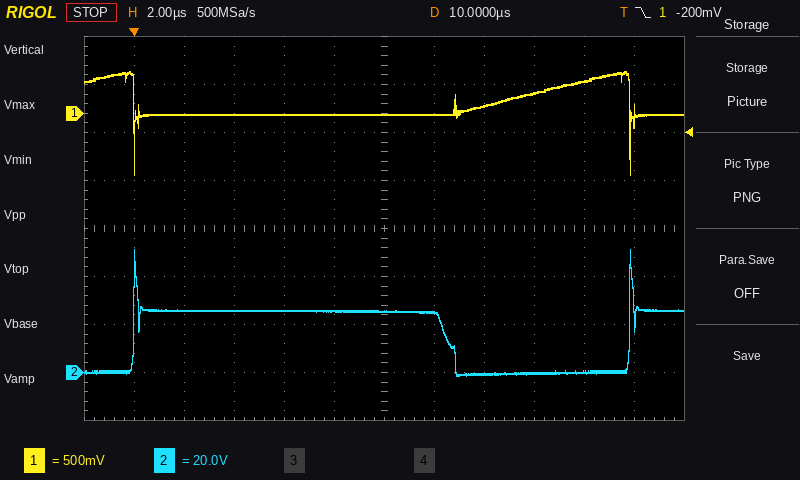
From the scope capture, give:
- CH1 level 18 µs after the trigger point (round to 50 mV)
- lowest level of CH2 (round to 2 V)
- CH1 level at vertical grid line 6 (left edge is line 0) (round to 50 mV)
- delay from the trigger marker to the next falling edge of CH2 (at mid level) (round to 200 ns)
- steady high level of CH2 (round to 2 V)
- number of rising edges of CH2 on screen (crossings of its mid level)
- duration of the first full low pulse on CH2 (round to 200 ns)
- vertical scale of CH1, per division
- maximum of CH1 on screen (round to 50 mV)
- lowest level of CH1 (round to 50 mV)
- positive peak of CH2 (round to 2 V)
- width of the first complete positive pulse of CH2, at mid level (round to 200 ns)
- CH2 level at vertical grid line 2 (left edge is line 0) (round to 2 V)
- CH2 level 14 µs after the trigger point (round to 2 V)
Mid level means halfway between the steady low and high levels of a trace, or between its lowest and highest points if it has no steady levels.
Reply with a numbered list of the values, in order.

1. 350 mV
2. -2 V
3. 0 mV
4. 12.6 µs
5. 26 V
6. 2
7. 7.2 µs
8. 500 mV
9. 450 mV
10. -650 mV
11. 52 V
12. 12.6 µs
13. 26 V
14. 0 V
